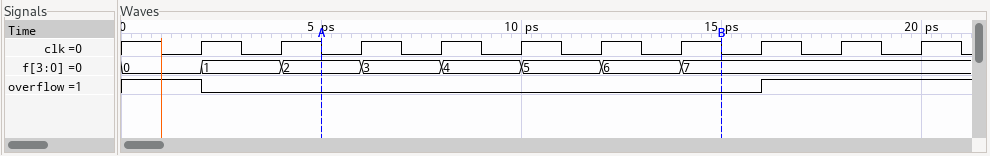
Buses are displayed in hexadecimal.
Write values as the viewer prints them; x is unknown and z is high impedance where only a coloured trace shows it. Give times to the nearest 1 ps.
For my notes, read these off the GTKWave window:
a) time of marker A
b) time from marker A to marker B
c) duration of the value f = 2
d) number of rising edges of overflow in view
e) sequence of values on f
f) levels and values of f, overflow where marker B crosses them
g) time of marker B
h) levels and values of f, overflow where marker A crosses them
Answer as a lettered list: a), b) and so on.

a) 5 ps
b) 10 ps
c) 2 ps
d) 1
e) 0, 1, 2, 3, 4, 5, 6, 7
f) f=7, overflow=0
g) 15 ps
h) f=2, overflow=0
